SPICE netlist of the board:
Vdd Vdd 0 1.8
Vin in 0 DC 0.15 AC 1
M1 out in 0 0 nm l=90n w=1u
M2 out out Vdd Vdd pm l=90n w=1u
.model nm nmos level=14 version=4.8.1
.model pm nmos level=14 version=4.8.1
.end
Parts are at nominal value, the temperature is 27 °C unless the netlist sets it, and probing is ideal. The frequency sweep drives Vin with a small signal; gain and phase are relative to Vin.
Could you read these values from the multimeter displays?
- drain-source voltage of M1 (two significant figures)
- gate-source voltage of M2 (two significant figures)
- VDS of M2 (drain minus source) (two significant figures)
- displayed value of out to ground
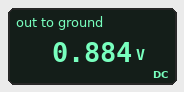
880 mV
-920 mV
-920 mV
0.884 V
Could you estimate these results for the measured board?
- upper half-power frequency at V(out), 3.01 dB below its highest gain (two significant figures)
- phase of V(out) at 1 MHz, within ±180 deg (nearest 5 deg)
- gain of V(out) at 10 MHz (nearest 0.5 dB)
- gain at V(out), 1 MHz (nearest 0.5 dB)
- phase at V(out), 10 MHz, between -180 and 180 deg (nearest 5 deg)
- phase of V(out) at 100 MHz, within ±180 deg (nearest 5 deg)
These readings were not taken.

5.0 MHz
170 deg
12.0 dB
18.5 dB
115 deg
60 deg
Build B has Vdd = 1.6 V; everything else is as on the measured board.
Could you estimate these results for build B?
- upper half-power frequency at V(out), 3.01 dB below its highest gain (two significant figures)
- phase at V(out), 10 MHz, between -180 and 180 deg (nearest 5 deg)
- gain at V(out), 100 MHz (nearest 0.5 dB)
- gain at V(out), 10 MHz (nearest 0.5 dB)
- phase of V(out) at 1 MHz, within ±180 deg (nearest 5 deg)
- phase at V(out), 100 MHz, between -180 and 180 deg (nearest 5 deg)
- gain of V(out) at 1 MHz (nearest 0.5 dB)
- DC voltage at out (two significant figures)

6.4 MHz
120 deg
-7.5 dB
9.5 dB
170 deg
55 deg
14.5 dB
760 mV
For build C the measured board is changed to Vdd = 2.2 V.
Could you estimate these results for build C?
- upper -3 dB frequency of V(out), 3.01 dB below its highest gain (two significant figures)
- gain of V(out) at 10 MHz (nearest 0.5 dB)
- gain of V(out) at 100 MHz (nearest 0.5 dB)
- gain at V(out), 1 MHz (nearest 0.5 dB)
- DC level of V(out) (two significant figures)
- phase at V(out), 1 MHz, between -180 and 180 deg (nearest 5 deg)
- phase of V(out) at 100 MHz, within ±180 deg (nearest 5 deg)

4.8 MHz
14.5 dB
-4.0 dB
21.5 dB
1.1 V
170 deg
70 deg
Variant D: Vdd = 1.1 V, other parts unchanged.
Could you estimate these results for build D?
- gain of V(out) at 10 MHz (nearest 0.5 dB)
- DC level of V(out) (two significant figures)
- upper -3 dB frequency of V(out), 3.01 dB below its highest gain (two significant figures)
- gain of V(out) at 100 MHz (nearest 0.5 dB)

1.0 dB
350 mV
6.7 MHz
-11.5 dB
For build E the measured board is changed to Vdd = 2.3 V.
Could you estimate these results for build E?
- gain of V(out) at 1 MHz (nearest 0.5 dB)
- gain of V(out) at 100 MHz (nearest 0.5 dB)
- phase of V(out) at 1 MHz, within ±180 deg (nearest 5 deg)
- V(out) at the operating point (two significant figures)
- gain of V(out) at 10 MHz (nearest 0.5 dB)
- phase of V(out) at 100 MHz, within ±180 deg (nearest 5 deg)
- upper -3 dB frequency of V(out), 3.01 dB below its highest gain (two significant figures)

22.0 dB
-3.5 dB
170 deg
1.1 V
15.0 dB
70 deg
4.9 MHz
